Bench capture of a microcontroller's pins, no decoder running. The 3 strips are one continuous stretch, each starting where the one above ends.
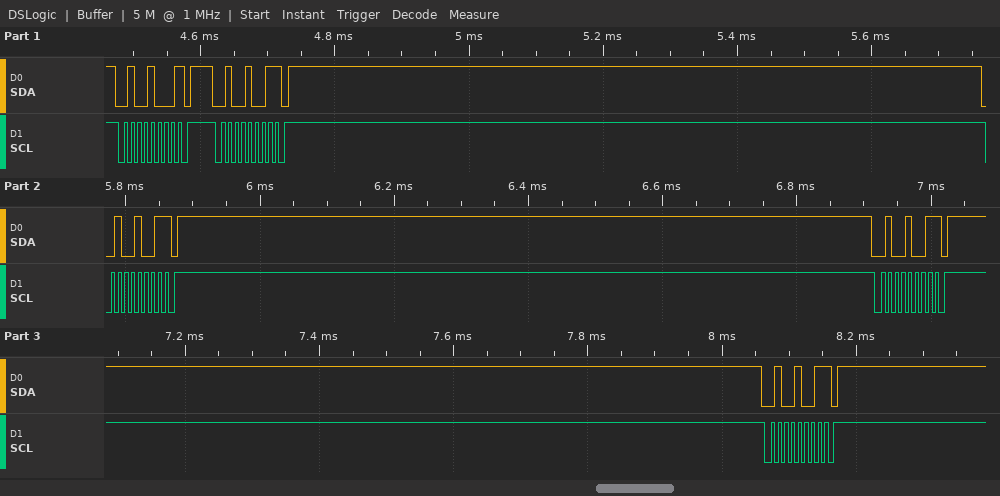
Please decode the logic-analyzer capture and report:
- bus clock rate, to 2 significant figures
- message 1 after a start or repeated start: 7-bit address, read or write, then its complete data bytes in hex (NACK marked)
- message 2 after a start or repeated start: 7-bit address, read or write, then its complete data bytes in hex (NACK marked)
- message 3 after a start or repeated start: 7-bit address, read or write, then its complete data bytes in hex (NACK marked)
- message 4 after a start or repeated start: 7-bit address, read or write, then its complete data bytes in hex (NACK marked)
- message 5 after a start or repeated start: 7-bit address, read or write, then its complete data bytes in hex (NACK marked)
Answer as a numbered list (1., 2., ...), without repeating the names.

1. 100 kHz
2. 0x24 write NACK
3. 0x24 read NACK
4. 0x24 read NACK
5. 0x24 read NACK
6. 0x24 read NACK
